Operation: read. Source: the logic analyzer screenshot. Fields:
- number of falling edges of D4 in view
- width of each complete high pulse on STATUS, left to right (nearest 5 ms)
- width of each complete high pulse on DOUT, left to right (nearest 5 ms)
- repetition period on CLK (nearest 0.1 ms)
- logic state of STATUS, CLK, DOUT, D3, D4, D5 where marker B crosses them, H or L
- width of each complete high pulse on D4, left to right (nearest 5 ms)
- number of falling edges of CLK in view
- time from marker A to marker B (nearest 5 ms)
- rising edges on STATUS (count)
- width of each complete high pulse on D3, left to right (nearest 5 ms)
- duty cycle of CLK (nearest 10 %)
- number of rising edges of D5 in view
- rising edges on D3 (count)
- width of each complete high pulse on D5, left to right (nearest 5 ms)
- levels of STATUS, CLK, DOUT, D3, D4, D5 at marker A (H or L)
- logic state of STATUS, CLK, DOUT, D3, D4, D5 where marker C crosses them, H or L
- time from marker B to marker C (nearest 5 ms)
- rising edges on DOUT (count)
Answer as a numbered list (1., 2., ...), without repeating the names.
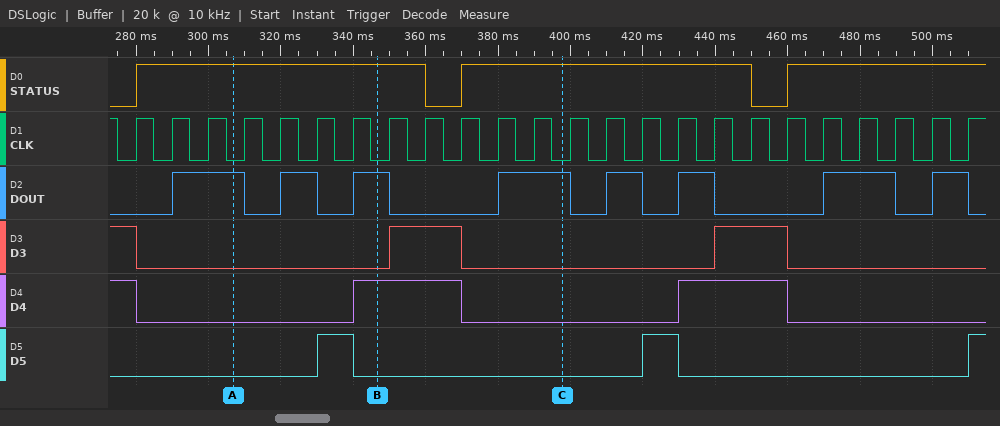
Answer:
1. 3
2. 80 ms, 80 ms
3. 20 ms, 10 ms, 10 ms, 20 ms, 10 ms, 10 ms, 20 ms, 10 ms
4. 10 ms
5. STATUS=H, CLK=L, DOUT=H, D3=L, D4=H, D5=L
6. 30 ms, 30 ms
7. 24
8. 40 ms
9. 3
10. 20 ms, 20 ms
11. 50 %
12. 3
13. 2
14. 10 ms, 10 ms
15. STATUS=H, CLK=L, DOUT=H, D3=L, D4=L, D5=L
16. STATUS=H, CLK=L, DOUT=H, D3=L, D4=L, D5=L
17. 50 ms
18. 8
